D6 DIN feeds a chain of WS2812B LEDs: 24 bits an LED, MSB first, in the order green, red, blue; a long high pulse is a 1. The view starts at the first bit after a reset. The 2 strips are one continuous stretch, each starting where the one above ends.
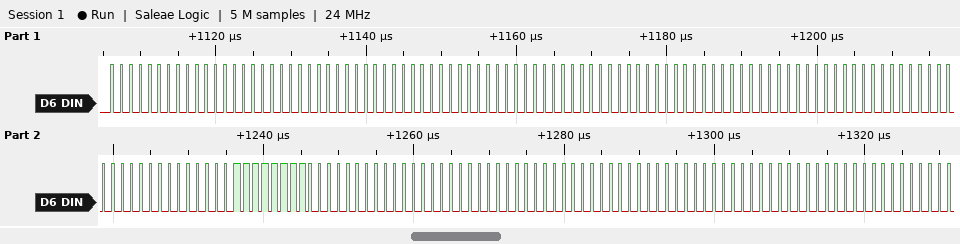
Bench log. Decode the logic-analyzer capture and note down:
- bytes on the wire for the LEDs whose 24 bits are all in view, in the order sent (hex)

00 00 00 00 00 00 00 00 00 00 00 00 00 FF 00 00 00 00 00 00 00
